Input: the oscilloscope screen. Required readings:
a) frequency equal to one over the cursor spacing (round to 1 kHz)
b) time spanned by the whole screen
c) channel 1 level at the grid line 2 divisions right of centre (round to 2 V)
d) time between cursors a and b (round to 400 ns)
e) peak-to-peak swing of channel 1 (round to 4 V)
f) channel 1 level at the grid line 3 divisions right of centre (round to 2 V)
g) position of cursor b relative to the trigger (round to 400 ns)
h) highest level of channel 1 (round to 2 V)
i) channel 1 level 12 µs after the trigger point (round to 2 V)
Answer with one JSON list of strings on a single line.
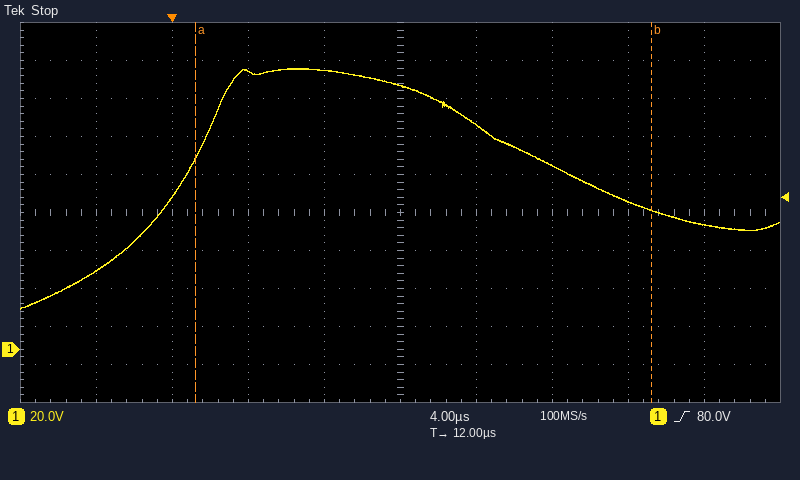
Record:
["42 kHz", "40 µs", "96 V", "24.0 µs", "128 V", "78 V", "+25.2 µs", "148 V", "138 V"]
